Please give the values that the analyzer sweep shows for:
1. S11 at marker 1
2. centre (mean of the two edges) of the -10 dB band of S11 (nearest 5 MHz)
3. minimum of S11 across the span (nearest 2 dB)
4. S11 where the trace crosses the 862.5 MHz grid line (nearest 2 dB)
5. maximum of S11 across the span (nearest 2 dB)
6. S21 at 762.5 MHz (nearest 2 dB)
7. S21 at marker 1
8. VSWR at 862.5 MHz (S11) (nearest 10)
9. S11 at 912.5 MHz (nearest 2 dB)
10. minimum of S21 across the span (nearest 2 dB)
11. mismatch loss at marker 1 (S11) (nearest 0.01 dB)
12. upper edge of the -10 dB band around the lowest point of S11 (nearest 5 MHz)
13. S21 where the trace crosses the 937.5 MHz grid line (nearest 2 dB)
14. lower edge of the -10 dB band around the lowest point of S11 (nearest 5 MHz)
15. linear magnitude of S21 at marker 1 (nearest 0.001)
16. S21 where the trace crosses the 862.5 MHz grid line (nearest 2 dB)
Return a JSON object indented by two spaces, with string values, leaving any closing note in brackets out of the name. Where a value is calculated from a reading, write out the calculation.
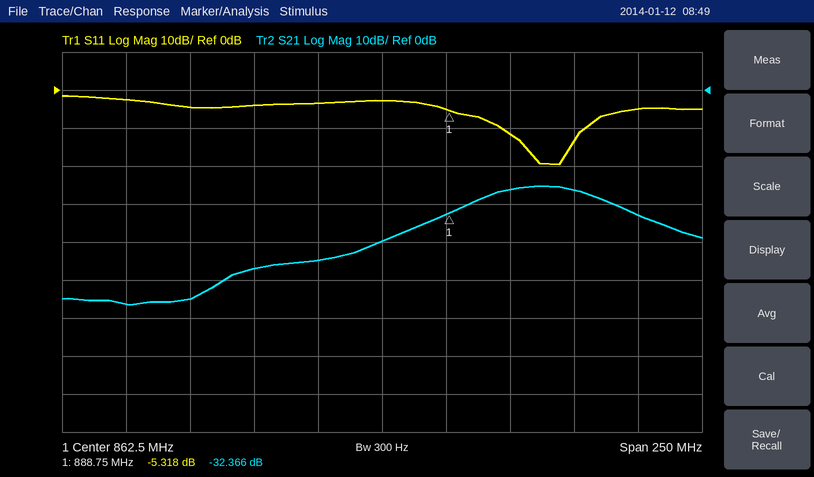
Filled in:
{
  "S11 at marker 1": "-5.318 dB",
  "centre (mean of the two edges) of the -10 dB band of S11": "925 MHz",
  "minimum of S11 across the span": "-20 dB",
  "S11 where the trace crosses the 862.5 MHz grid line": "-2 dB",
  "maximum of S11 across the span": "-2 dB",
  "S21 at 762.5 MHz": "-56 dB",
  "S21 at marker 1": "-32.366 dB",
  "VSWR at 862.5 MHz (S11)": "|Γ| = 10^(-2/20) = 0.7943; VSWR = (1 + 0.7943)/(1 − 0.7943) ≈ 8.72, so 10 to the nearest 10",
  "S11 at 912.5 MHz": "-12 dB",
  "minimum of S21 across the span": "-56 dB",
  "mismatch loss at marker 1 (S11)": "−10 log10(1 − 10^(-5.318/10)) ≈ 1.51 dB",
  "upper edge of the -10 dB band around the lowest point of S11": "940 MHz",
  "S21 where the trace crosses the 937.5 MHz grid line": "-26 dB",
  "lower edge of the -10 dB band around the lowest point of S11": "910 MHz",
  "linear magnitude of S21 at marker 1": "10^(-32.366/20) ≈ 0.024",
  "S21 where the trace crosses the 862.5 MHz grid line": "-40 dB"
}
